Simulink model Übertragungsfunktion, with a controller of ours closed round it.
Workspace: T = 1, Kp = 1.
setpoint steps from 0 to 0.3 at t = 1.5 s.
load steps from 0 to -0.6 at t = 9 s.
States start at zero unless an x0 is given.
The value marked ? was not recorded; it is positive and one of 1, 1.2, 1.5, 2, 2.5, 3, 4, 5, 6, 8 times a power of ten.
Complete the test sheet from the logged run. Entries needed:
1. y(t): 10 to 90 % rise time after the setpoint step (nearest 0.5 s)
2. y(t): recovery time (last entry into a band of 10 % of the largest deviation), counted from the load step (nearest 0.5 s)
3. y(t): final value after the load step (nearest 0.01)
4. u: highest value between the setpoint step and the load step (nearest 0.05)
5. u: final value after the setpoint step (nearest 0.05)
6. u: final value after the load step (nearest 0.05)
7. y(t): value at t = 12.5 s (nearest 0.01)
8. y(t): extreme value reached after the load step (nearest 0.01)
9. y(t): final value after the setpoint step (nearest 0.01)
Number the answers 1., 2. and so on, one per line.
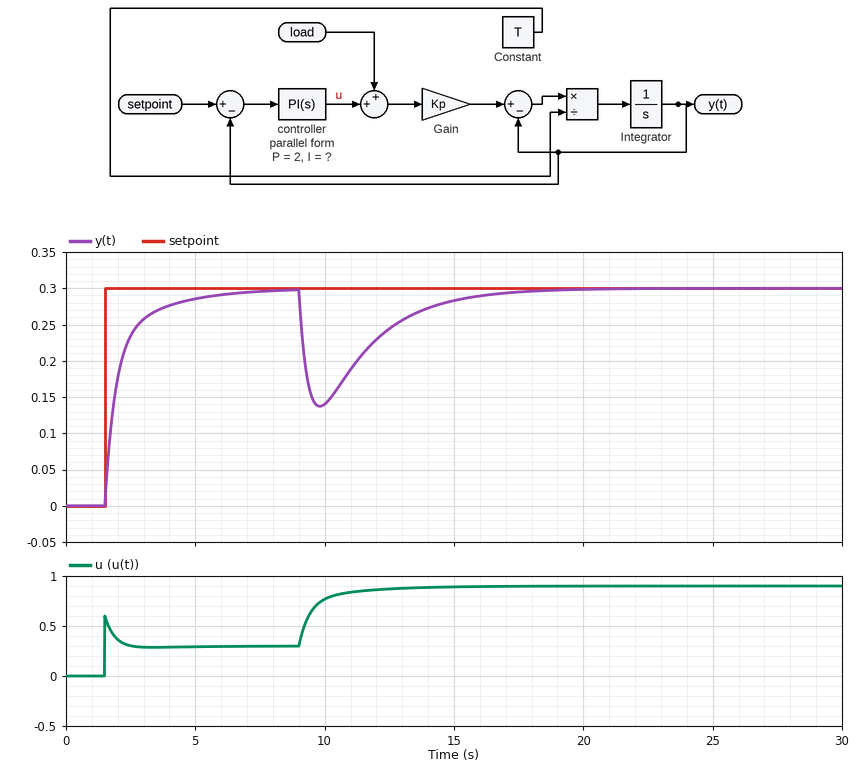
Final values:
1. 2.0 s
2. 6.0 s
3. 0.30
4. 0.60
5. 0.30
6. 0.90
7. 0.24
8. 0.14
9. 0.30
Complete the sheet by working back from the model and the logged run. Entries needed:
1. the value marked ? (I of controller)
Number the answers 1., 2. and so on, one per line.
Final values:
1. 1.2
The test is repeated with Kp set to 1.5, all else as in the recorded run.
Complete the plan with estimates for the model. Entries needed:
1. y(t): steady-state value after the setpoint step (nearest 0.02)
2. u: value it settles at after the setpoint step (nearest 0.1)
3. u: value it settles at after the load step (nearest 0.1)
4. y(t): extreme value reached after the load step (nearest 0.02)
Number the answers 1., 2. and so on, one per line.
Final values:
1. 0.30
2. 0.2
3. 0.8
4. 0.12
